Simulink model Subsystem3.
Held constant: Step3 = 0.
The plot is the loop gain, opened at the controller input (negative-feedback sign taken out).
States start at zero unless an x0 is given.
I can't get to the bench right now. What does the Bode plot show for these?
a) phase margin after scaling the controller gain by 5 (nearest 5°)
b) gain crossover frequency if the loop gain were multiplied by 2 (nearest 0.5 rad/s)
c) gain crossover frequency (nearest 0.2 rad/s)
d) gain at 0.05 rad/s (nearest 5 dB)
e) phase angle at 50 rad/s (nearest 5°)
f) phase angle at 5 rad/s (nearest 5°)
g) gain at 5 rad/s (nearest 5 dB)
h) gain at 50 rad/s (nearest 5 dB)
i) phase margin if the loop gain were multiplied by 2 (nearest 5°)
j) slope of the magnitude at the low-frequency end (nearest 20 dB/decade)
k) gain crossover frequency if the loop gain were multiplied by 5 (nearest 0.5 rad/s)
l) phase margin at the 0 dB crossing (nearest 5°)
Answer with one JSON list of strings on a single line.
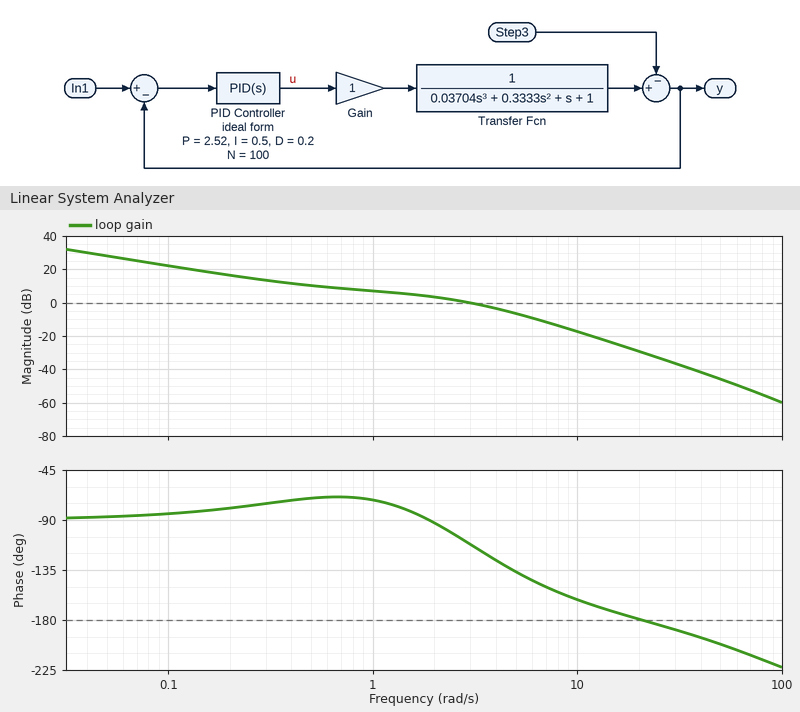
["25°", "5.0 rad/s", "3.0 rad/s", "30 dB", "-200°", "-135°", "-5 dB", "-45 dB", "45°", "-20 dB/decade", "8.0 rad/s", "70°"]
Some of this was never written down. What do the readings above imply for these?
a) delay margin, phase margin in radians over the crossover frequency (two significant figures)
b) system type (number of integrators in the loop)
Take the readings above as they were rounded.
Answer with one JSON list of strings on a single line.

["0.41 s", "1"]
